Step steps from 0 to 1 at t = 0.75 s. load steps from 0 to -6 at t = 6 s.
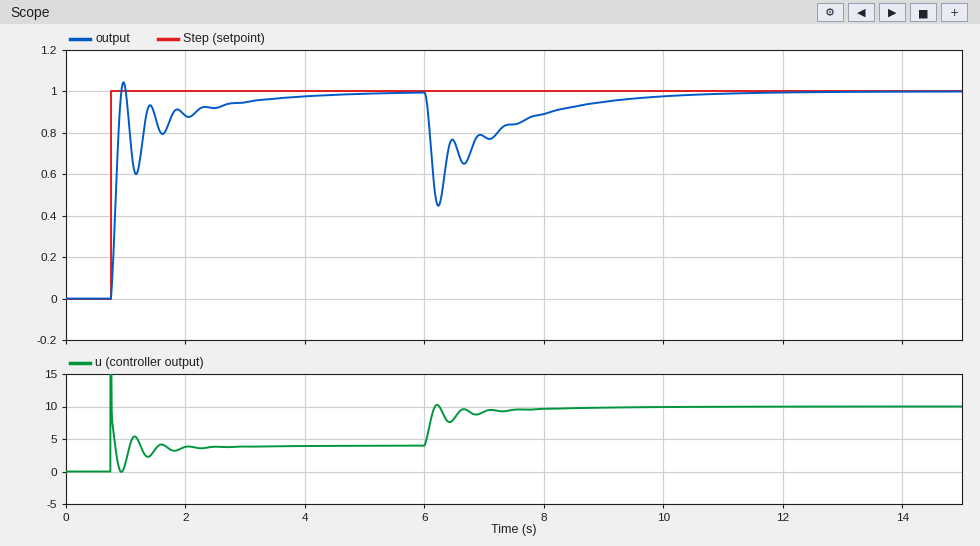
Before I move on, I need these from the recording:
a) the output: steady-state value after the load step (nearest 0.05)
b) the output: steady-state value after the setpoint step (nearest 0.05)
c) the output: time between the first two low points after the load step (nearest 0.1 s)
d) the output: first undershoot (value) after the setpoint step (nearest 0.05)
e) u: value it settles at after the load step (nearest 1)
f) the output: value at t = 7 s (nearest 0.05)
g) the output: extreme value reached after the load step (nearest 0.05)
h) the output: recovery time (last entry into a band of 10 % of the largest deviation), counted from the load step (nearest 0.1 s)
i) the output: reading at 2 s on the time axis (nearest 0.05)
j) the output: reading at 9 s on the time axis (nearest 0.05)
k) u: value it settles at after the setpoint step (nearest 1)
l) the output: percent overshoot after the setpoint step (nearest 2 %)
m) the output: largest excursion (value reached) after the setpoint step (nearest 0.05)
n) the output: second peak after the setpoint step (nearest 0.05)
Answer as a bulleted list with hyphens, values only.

- 1.00
- 1.00
- 0.4 s
- 0.60
- 10
- 0.80
- 0.45
- 2.9 s
- 0.90
- 0.95
- 4
- 4 %
- 1.05
- 0.95
